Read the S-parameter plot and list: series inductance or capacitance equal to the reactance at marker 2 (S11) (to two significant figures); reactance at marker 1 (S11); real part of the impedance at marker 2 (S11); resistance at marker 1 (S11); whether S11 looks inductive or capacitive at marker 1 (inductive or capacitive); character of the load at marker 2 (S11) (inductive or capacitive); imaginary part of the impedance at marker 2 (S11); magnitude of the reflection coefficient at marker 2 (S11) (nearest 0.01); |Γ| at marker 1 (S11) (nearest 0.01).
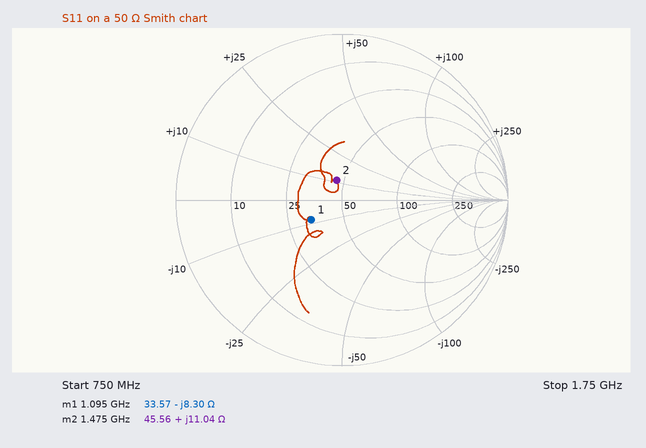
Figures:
1.2 nH
-8.30 Ω
45.56 Ω
33.57 Ω
capacitive
inductive
+11.04 Ω
0.12
0.22
